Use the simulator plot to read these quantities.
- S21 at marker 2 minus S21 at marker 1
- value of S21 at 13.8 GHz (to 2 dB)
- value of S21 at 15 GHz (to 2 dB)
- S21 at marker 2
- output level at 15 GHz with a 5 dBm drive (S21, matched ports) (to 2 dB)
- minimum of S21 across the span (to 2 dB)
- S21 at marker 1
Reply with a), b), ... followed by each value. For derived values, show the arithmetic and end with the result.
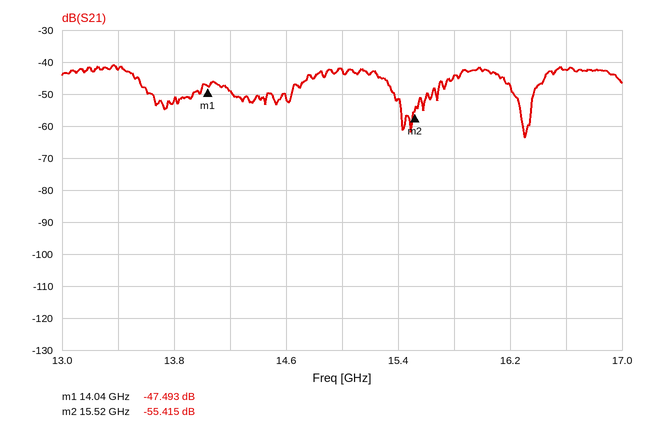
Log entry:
a) -55.415 − (-47.493) = -7.922 dB
b) -52 dB
c) -42 dB
d) -55.415 dB
e) 5 dBm + (-42 dB) = -38 dBm
f) -64 dB
g) -47.493 dB
